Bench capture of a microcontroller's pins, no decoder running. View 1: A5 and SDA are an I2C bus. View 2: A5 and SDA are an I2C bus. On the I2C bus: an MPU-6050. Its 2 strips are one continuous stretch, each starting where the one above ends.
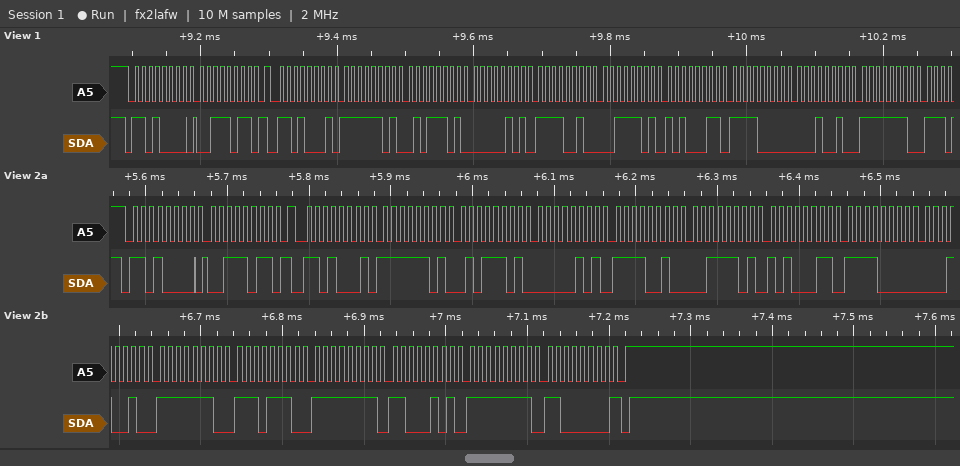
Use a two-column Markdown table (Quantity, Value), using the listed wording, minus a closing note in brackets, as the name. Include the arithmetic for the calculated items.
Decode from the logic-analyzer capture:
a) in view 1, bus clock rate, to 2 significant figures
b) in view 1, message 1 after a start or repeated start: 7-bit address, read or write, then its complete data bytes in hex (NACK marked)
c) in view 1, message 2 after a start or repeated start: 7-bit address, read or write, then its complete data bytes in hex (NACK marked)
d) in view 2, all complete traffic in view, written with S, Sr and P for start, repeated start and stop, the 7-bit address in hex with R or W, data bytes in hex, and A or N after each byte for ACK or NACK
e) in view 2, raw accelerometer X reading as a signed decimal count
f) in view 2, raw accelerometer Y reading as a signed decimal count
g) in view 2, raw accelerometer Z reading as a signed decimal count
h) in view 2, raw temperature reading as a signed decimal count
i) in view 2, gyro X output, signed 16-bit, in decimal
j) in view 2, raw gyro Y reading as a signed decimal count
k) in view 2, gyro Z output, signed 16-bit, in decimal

| Quantity | Value |
|---|---|
| in view 1, bus clock rate, to 2 significant figures | 100 kHz |
| in view 1, message 1 after a start or repeated start: 7-bit address, read or write, then its complete data bytes in hex | 0x68 write: 3B |
| in view 1, message 2 after a start or repeated start: 7-bit address, read or write, then its complete data bytes in hex | 0x68 read: FD 5D 05 F2 3D A3 F0 12 FE |
| in view 2, all complete traffic in view, written with S, Sr and P for start, repeated start and stop, the 7-bit address in hex with R or W, data bytes in hex, and A or N after each byte for ACK or NACK | S 68W A 3B A Sr 68R A FD A 5D A 05 A F2 A 3D A A3 A F0 A 12 A FE A EE A FF A C5 A FF A C0 N P |
| in view 2, raw accelerometer X reading as a signed decimal count | 0xFD5D = -675 |
| in view 2, raw accelerometer Y reading as a signed decimal count | 0x05F2 = 1522 |
| in view 2, raw accelerometer Z reading as a signed decimal count | 0x3DA3 = 15779 |
| in view 2, raw temperature reading as a signed decimal count | 0xF012 = -4078 |
| in view 2, gyro X output, signed 16-bit, in decimal | 0xFEEE = -274 |
| in view 2, raw gyro Y reading as a signed decimal count | 0xFFC5 = -59 |
| in view 2, gyro Z output, signed 16-bit, in decimal | 0xFFC0 = -64 |
